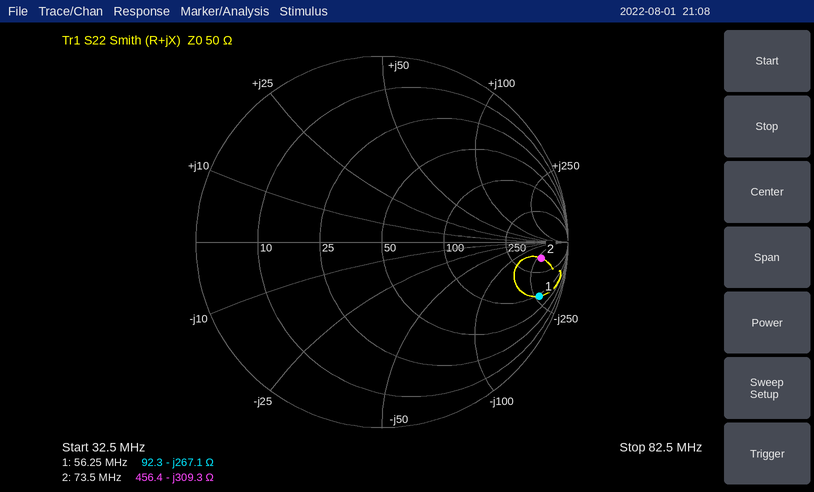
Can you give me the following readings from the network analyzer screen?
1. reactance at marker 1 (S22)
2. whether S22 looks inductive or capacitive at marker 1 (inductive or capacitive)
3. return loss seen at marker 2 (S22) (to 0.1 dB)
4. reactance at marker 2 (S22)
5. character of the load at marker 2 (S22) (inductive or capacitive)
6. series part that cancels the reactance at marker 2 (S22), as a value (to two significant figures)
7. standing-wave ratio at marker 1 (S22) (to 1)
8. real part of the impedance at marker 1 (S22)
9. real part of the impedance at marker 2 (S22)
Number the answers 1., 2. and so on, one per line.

1. -267.1 Ω
2. capacitive
3. 1.3 dB
4. -309.3 Ω
5. capacitive
6. 670 nH
7. 18
8. 92.3 Ω
9. 456.4 Ω
